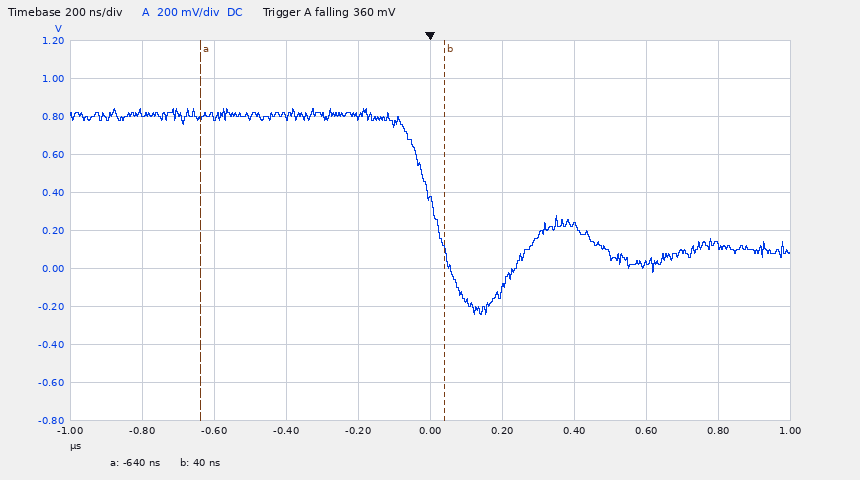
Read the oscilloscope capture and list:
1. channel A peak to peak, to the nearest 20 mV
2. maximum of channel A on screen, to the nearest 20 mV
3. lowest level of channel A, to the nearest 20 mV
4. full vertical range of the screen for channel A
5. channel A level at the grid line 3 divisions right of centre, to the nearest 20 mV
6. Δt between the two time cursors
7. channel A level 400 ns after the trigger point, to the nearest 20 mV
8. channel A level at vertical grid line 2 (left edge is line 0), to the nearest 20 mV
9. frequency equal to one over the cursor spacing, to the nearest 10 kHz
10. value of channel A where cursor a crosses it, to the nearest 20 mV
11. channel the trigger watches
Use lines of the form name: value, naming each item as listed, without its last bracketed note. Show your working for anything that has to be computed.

channel A peak to peak, to the nearest 20 mV: 840 mV − (-240 mV) = 1.08 V
maximum of channel A on screen, to the nearest 20 mV: 840 mV
lowest level of channel A, to the nearest 20 mV: -240 mV
full vertical range of the screen for channel A: 2 V
channel A level at the grid line 3 divisions right of centre, to the nearest 20 mV: 20 mV
Δt between the two time cursors: 40 ns − (-640 ns) = 680 ns
channel A level 400 ns after the trigger point, to the nearest 20 mV: 220 mV
channel A level at vertical grid line 2 (left edge is line 0), to the nearest 20 mV: 800 mV
frequency equal to one over the cursor spacing, to the nearest 10 kHz: 1 / 680 ns ≈ 1.47 MHz
value of channel A where cursor a crosses it, to the nearest 20 mV: 800 mV
channel the trigger watches: channel A
